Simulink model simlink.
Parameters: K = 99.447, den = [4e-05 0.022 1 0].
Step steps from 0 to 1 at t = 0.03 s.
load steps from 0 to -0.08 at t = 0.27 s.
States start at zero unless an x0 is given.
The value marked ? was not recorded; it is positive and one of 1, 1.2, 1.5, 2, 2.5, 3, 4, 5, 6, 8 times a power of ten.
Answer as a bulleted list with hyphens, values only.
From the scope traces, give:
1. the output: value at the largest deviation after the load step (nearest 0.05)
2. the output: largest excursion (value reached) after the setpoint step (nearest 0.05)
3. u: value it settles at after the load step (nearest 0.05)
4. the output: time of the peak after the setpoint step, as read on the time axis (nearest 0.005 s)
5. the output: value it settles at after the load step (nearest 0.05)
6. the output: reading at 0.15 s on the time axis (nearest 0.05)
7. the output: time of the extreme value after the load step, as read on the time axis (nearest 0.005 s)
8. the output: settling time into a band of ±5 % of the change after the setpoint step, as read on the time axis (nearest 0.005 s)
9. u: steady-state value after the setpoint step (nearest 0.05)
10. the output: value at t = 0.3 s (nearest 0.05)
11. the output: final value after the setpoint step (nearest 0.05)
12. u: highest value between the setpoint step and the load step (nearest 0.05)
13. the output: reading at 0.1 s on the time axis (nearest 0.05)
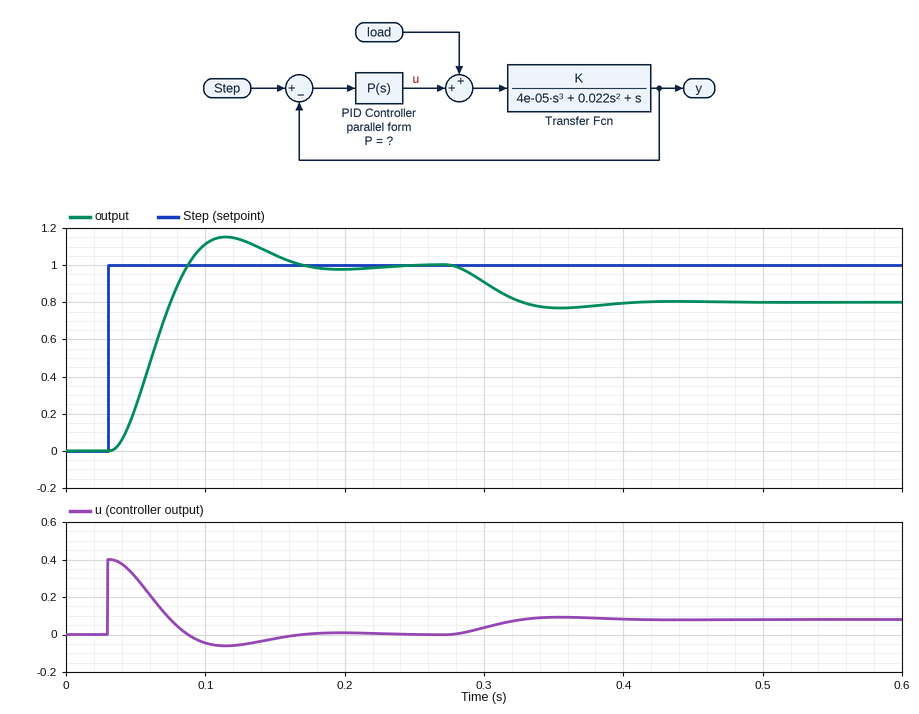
- 0.75
- 1.15
- 0.10
- 0.115 s
- 0.80
- 1.05
- 0.355 s
- 0.150 s
- 0.00
- 0.90
- 1.00
- 0.40
- 1.10
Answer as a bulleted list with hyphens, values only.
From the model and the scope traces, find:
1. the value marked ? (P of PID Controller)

- 0.4
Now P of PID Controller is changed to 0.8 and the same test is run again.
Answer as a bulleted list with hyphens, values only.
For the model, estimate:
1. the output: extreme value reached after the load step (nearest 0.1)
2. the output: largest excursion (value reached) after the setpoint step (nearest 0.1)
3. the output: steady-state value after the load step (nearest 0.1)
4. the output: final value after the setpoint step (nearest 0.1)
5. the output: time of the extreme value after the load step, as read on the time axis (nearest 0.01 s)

- 0.9
- 1.3
- 0.9
- 1.0
- 0.33 s
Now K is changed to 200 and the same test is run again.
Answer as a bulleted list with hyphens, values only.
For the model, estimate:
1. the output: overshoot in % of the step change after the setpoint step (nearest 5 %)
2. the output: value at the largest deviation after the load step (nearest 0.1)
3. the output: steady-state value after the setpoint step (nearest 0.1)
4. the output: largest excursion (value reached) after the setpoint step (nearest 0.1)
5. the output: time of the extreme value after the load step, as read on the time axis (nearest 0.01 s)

- 35 %
- 0.7
- 1.0
- 1.3
- 0.33 s
